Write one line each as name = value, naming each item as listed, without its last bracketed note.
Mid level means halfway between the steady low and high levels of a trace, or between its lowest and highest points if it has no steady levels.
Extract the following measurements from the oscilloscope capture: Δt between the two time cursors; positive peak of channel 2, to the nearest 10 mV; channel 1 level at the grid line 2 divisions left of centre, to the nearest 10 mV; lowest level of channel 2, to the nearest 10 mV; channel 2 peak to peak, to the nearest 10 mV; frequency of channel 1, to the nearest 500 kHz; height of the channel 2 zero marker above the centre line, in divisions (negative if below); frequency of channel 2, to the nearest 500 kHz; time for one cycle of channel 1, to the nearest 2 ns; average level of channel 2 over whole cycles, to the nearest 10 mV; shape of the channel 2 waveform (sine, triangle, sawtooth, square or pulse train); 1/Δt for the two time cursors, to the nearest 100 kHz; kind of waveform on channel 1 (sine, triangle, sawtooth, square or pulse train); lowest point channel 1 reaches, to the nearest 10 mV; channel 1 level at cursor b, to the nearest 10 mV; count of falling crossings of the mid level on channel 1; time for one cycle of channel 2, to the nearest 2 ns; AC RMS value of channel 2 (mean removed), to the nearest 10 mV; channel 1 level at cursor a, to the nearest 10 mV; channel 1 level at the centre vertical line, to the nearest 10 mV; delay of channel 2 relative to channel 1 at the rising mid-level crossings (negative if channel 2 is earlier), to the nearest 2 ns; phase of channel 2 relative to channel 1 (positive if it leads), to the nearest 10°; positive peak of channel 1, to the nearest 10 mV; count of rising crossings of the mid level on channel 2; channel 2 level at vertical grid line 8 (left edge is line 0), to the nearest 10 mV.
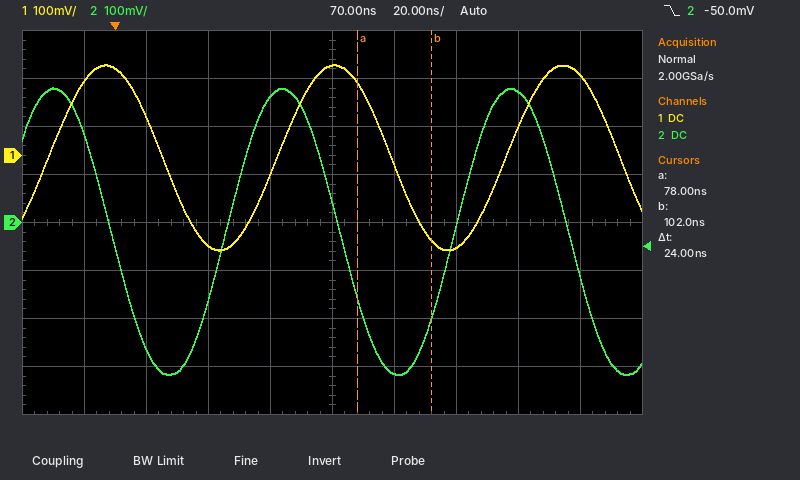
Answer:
Δt between the two time cursors = 24 ns
positive peak of channel 2, to the nearest 10 mV = 280 mV
channel 1 level at the grid line 2 divisions left of centre, to the nearest 10 mV = -190 mV
lowest level of channel 2, to the nearest 10 mV = -320 mV
channel 2 peak to peak, to the nearest 10 mV = 600 mV
frequency of channel 1, to the nearest 500 kHz = 13.5 MHz
height of the channel 2 zero marker above the centre line, in divisions = 0.0 div
frequency of channel 2, to the nearest 500 kHz = 13.5 MHz
time for one cycle of channel 1, to the nearest 2 ns = 74 ns
average level of channel 2 over whole cycles, to the nearest 10 mV = -20 mV
shape of the channel 2 waveform = sine
1/Δt for the two time cursors, to the nearest 100 kHz = 41.7 MHz
kind of waveform on channel 1 = sine
lowest point channel 1 reaches, to the nearest 10 mV = -200 mV
channel 1 level at cursor b, to the nearest 10 mV = -180 mV
count of falling crossings of the mid level on channel 1 = 3
time for one cycle of channel 2, to the nearest 2 ns = 74 ns
AC RMS value of channel 2 (mean removed), to the nearest 10 mV = 210 mV
channel 1 level at cursor a, to the nearest 10 mV = 150 mV
channel 1 level at the centre vertical line, to the nearest 10 mV = 190 mV
delay of channel 2 relative to channel 1 at the rising mid-level crossings (negative if channel 2 is earlier), to the nearest 2 ns = -16 ns
phase of channel 2 relative to channel 1 (positive if it leads), to the nearest 10° = +80°
positive peak of channel 1, to the nearest 10 mV = 190 mV
count of rising crossings of the mid level on channel 2 = 2
channel 2 level at vertical grid line 8 (left edge is line 0), to the nearest 10 mV = 270 mV
